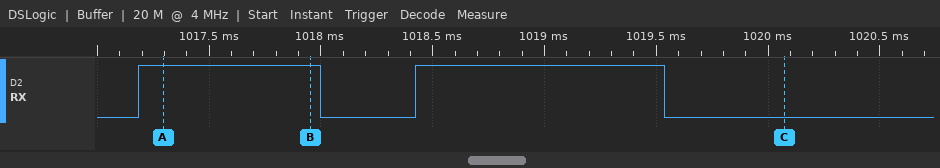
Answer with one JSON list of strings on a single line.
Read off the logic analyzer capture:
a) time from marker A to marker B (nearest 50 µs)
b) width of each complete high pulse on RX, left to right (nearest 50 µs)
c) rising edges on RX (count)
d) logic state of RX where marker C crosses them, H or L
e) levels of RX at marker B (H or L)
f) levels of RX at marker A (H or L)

["650 µs", "800 µs, 1100 µs", "2", "RX=L", "RX=H", "RX=H"]
